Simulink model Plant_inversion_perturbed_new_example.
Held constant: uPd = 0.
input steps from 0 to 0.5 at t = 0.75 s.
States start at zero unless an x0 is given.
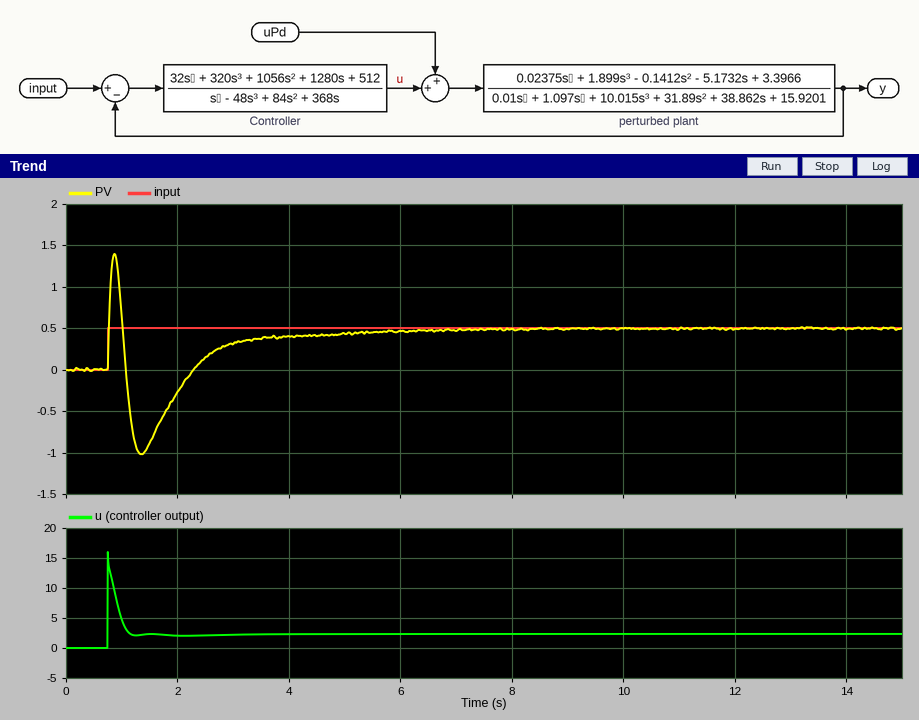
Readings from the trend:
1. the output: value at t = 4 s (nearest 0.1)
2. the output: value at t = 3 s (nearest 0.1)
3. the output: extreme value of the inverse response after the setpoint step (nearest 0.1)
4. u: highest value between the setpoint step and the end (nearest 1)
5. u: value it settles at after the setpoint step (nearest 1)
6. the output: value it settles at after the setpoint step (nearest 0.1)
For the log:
0.4
0.3
-1.0
16
2
0.5
